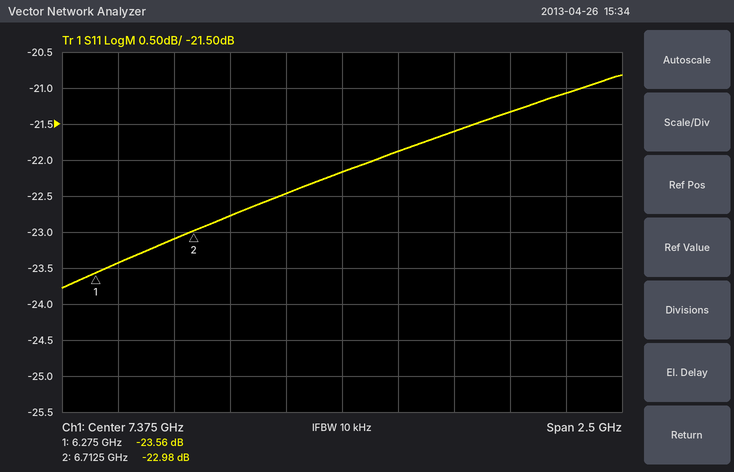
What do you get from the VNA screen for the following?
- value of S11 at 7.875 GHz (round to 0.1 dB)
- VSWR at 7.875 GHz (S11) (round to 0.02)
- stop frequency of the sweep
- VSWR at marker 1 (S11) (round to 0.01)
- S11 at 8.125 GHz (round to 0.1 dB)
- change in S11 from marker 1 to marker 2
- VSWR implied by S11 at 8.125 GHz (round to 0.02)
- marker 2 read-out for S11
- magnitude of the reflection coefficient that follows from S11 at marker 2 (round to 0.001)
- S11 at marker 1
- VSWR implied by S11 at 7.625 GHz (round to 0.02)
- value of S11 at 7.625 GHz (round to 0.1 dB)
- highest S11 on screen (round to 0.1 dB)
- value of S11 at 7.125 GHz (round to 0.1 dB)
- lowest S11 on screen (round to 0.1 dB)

-21.6 dB
1.18
8.625 GHz
1.14
-21.3 dB
0.58 dB
1.18
-22.98 dB
0.071
-23.56 dB
1.18
-21.9 dB
-20.8 dB
-22.5 dB
-23.8 dB
